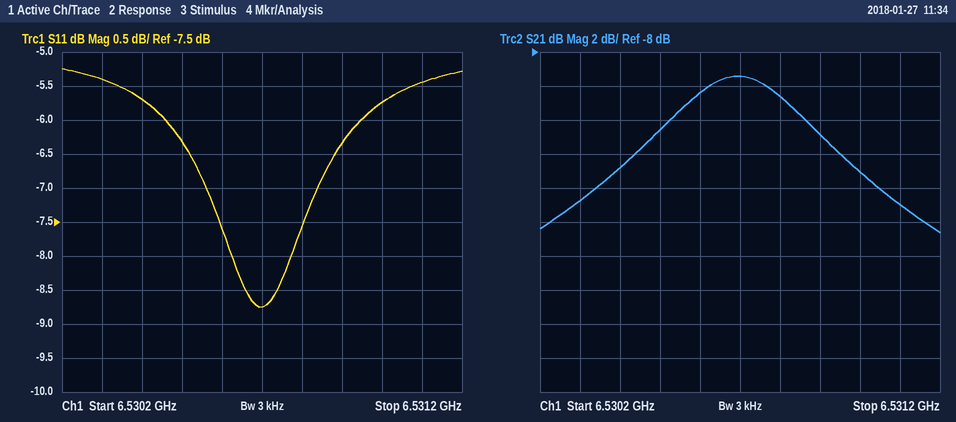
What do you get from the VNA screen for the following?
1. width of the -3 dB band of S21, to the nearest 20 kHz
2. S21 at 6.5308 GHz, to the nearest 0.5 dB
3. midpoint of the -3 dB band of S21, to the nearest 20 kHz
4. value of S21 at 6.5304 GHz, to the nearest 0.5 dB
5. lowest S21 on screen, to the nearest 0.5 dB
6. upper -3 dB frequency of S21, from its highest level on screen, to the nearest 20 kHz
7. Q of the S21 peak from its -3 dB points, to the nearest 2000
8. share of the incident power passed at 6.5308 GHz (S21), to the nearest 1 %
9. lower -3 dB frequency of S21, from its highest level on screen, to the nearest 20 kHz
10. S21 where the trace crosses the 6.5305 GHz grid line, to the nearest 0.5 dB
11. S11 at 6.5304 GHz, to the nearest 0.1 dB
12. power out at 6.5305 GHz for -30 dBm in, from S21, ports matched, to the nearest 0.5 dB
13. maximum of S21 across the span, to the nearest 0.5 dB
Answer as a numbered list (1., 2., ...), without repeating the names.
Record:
1. 380 kHz
2. -10.5 dB
3. 6.53070 GHz
4. -15.0 dB
5. -18.5 dB
6. 6.53088 GHz
7. 18000
8. 9 %
9. 6.53050 GHz
10. -12.5 dB
11. -5.7 dB
12. -42.5 dBm
13. -9.5 dB
